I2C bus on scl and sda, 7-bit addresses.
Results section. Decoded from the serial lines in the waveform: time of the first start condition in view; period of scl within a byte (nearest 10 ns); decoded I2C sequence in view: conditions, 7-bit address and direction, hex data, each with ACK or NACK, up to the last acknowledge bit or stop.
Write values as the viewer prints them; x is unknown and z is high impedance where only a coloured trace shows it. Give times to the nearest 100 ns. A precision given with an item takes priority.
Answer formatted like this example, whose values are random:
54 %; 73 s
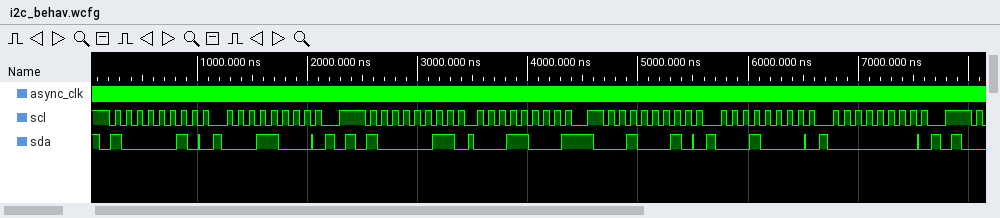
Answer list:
100 ns; 100 ns; start, address 41 write ACK, 18 ACK, stop, start, address 41 read ACK, 18 NACK, repeated start, address 11 write ACK, 10 ACK, 00 ACK, stop
